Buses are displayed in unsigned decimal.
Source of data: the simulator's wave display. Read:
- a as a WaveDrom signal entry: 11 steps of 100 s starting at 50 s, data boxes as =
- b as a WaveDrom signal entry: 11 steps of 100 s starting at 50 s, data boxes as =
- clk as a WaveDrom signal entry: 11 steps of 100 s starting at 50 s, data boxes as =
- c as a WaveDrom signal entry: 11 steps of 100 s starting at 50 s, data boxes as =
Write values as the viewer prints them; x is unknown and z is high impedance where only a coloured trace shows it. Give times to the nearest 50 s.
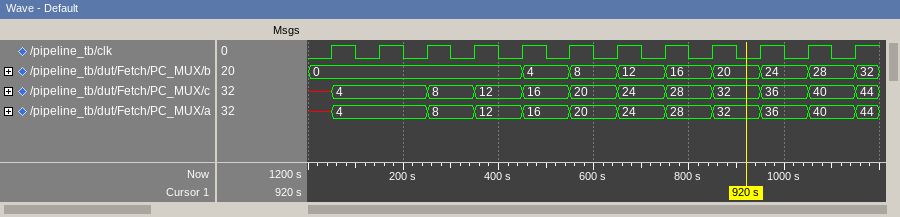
{name: 'a', wave: '=.=========', data: '4 8 12 16 20 24 28 32 36 40'}
{name: 'b', wave: '=...=======', data: '0 4 8 12 16 20 24 28'}
{name: 'clk', wave: 'p..........'}
{name: 'c', wave: '=.=========', data: '4 8 12 16 20 24 28 32 36 40'}
